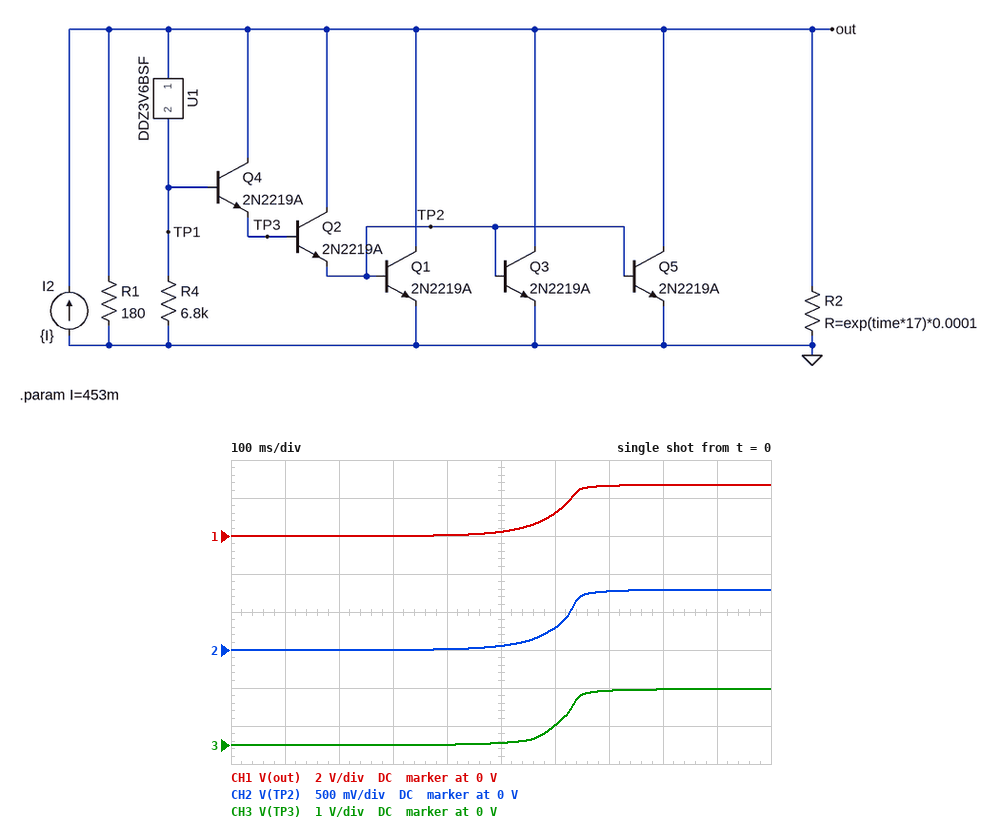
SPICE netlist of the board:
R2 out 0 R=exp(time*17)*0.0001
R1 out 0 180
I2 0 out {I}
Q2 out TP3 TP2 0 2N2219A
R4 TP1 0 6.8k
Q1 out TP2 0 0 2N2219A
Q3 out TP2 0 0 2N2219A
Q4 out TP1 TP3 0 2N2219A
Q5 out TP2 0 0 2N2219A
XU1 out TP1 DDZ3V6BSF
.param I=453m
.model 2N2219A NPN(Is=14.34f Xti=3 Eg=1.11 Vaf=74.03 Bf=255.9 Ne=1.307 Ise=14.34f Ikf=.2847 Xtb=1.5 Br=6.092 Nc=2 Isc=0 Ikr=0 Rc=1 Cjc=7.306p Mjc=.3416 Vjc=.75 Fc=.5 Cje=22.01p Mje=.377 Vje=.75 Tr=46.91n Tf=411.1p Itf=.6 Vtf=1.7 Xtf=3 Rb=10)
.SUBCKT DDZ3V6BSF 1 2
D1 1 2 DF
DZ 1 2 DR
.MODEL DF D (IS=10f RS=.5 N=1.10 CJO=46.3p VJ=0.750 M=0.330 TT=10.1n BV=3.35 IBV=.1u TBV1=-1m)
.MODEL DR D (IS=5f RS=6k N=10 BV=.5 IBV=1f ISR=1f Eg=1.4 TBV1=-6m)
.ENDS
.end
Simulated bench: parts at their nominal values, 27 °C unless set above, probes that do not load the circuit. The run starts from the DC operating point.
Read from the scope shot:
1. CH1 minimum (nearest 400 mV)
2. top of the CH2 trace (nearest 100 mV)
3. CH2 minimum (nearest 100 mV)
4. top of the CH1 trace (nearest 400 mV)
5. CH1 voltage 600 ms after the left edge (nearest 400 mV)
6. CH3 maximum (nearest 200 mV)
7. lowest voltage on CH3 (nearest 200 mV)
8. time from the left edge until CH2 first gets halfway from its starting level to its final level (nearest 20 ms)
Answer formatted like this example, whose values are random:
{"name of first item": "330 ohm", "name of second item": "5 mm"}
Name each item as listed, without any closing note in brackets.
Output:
{"CH1 minimum": "0 V", "top of the CH2 trace": "800 mV", "CH2 minimum": "0 V", "top of the CH1 trace": "2.8 V", "CH1 voltage 600 ms after the left edge": "1.2 V", "CH3 maximum": "1.4 V", "lowest voltage on CH3": "0 V", "time from the left edge until CH2 first gets halfway from its starting level to its final level": "620 ms"}
